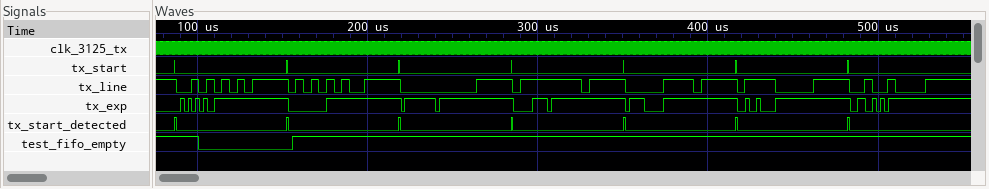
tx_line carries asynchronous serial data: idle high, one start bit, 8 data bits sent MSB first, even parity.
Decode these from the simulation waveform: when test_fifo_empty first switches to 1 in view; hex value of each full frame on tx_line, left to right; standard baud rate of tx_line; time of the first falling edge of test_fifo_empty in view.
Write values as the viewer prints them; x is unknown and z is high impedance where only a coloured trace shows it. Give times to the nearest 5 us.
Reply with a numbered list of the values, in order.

1. 155 us
2. 55, AA, 00, FF, 0F, F0, 48
3. 230400 baud
4. 100 us
